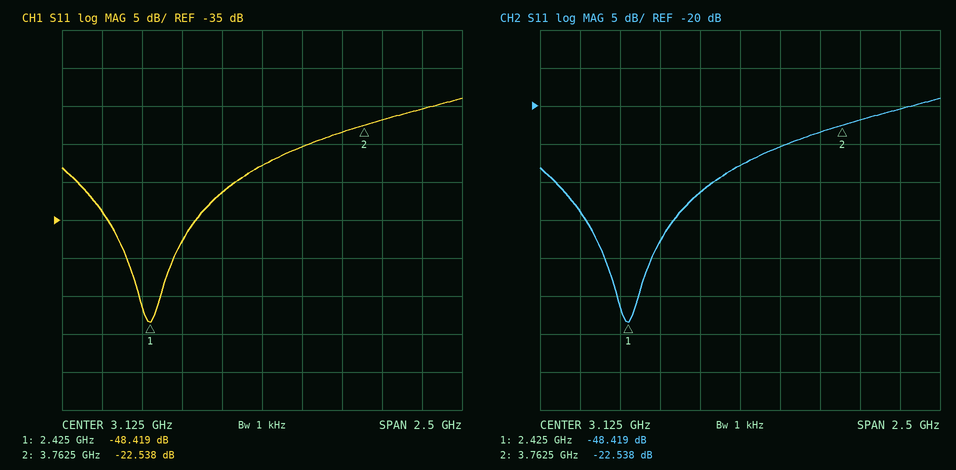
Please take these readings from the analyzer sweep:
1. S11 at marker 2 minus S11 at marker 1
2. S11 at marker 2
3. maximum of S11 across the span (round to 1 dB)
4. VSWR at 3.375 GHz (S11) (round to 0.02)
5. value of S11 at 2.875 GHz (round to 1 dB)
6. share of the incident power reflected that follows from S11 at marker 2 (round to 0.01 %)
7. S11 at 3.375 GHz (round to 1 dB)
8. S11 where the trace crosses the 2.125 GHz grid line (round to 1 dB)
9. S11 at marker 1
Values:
25.881 dB
-22.538 dB
-19 dB
1.12
-31 dB
0.56 %
-25 dB
-34 dB
-48.419 dB
